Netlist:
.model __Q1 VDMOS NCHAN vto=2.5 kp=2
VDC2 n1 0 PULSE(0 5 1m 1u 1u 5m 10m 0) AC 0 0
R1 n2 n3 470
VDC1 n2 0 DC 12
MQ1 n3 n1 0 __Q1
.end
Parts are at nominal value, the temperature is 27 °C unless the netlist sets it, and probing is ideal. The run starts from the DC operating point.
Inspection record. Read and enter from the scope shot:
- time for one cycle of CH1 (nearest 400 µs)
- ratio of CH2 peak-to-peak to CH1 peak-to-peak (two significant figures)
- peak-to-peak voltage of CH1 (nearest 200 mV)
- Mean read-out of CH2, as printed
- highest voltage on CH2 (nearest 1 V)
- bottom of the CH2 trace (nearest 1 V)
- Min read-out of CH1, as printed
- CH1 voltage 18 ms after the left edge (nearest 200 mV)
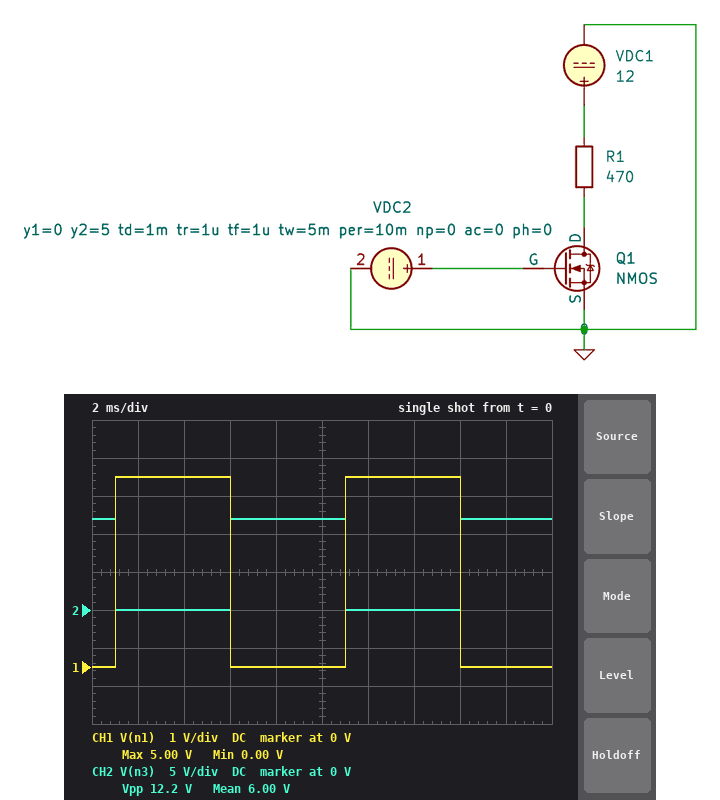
10.0 ms
2.4
5.0 V
6.00 V
12 V
0 V
0.00 V
0 V
